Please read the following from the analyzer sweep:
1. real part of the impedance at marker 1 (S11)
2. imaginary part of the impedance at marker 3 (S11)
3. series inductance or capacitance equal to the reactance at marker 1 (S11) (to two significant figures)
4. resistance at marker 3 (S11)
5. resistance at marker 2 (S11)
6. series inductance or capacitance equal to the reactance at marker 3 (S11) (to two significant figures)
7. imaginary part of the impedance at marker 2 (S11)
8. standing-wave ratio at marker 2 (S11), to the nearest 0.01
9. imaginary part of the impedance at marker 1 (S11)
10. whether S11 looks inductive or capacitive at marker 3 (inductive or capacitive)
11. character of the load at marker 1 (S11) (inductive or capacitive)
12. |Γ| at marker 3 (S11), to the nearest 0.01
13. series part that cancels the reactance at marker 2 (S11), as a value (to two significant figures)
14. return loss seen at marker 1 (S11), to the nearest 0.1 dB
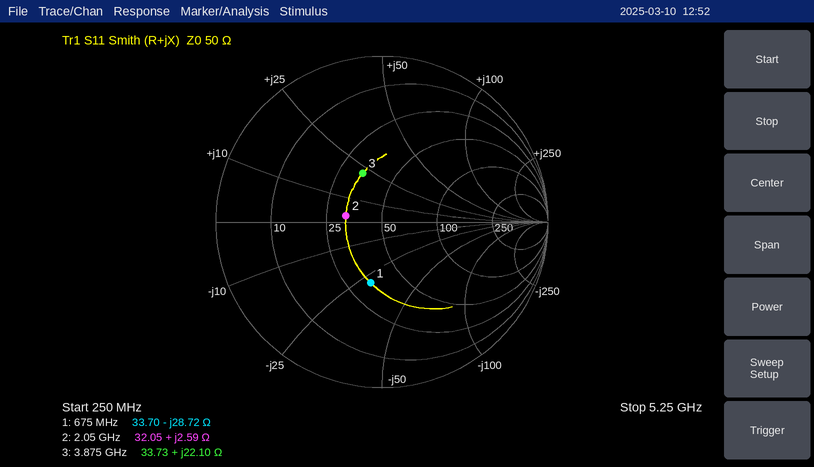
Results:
33.70 Ω
+22.10 Ω
8.2 pF
33.73 Ω
32.05 Ω
910 pH
+2.59 Ω
1.57
-28.72 Ω
inductive
capacitive
0.32
30 pF
8.6 dB
